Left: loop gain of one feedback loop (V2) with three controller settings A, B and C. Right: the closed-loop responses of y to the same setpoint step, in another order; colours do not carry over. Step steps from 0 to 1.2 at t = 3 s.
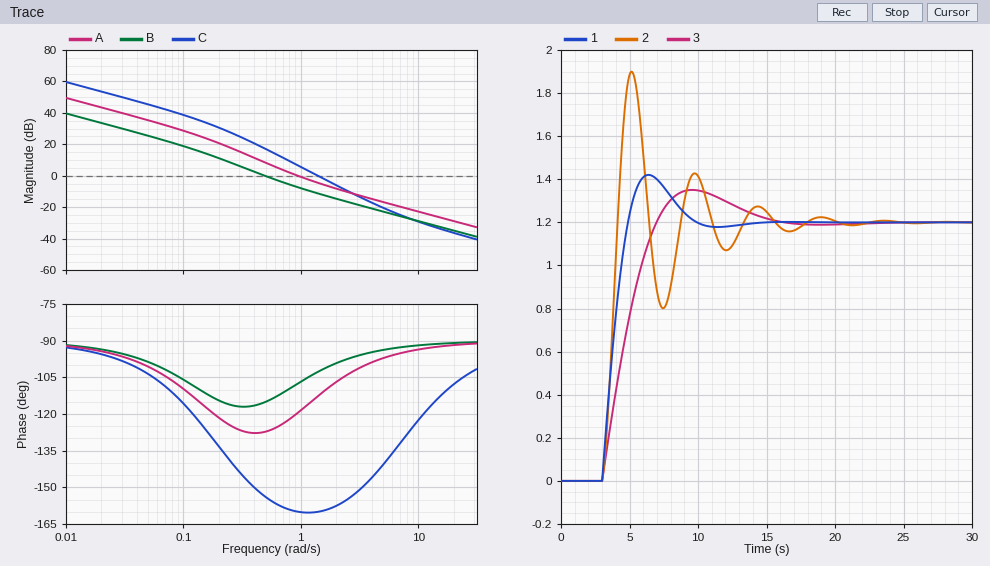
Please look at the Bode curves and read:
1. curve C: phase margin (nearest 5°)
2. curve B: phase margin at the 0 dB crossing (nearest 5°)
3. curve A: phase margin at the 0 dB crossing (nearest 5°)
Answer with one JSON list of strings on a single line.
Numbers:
["20°", "65°", "60°"]
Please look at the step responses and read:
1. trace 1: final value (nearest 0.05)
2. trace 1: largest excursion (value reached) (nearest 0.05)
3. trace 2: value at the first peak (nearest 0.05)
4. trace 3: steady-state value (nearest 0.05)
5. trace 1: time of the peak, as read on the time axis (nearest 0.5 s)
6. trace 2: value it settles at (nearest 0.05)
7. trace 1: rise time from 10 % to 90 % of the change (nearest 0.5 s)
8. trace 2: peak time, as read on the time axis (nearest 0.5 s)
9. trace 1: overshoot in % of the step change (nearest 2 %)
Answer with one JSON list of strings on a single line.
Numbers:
["1.20", "1.40", "1.90", "1.20", "6.5 s", "1.20", "1.5 s", "5.0 s", "18 %"]
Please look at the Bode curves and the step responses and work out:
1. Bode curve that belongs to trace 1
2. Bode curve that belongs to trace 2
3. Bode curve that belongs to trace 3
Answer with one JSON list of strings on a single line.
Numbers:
["A", "C", "B"]
